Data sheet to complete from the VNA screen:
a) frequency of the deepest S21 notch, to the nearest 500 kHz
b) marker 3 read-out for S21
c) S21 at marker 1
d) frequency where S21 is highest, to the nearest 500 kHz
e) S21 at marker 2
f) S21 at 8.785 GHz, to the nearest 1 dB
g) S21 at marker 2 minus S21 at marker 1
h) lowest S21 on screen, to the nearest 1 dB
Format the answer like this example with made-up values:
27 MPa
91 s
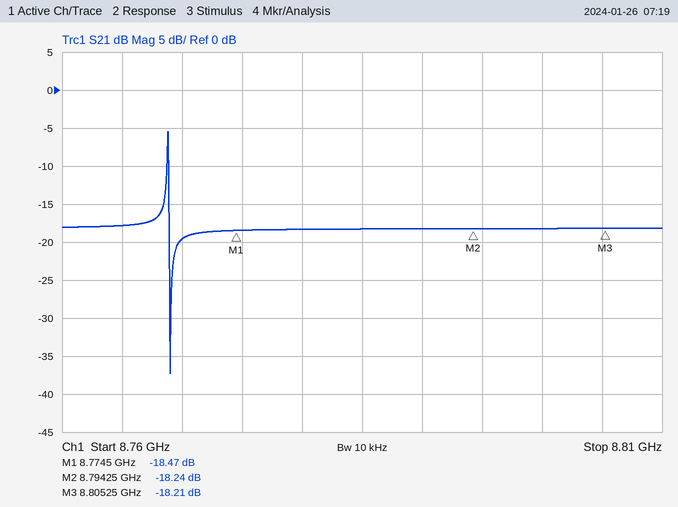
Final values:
8.7690 GHz
-18.21 dB
-18.47 dB
8.7690 GHz
-18.24 dB
-18 dB
0.23 dB
-37 dB
